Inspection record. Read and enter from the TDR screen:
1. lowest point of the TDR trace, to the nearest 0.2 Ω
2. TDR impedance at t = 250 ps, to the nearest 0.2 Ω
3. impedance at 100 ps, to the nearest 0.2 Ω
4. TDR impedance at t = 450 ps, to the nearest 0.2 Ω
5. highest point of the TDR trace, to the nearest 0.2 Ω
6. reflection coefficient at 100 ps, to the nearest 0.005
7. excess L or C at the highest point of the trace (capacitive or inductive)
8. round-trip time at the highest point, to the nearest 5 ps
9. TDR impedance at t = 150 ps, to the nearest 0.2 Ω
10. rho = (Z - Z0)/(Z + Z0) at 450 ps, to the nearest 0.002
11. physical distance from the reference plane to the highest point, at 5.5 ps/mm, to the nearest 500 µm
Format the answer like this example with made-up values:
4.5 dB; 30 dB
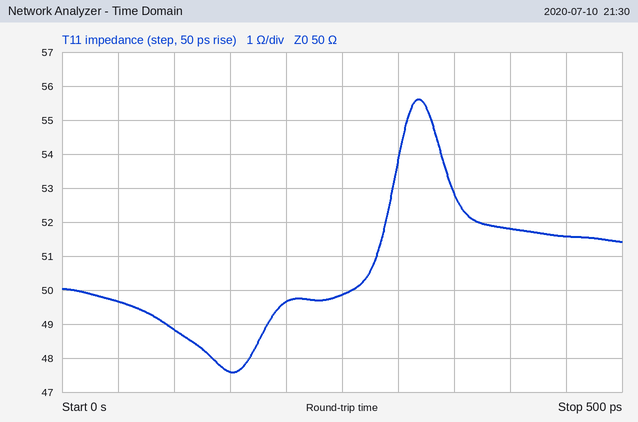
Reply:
47.6 Ω; 49.8 Ω; 48.8 Ω; 51.6 Ω; 55.6 Ω; -0.010; inductive; 320 ps; 47.6 Ω; +0.016; 29.0 mm
